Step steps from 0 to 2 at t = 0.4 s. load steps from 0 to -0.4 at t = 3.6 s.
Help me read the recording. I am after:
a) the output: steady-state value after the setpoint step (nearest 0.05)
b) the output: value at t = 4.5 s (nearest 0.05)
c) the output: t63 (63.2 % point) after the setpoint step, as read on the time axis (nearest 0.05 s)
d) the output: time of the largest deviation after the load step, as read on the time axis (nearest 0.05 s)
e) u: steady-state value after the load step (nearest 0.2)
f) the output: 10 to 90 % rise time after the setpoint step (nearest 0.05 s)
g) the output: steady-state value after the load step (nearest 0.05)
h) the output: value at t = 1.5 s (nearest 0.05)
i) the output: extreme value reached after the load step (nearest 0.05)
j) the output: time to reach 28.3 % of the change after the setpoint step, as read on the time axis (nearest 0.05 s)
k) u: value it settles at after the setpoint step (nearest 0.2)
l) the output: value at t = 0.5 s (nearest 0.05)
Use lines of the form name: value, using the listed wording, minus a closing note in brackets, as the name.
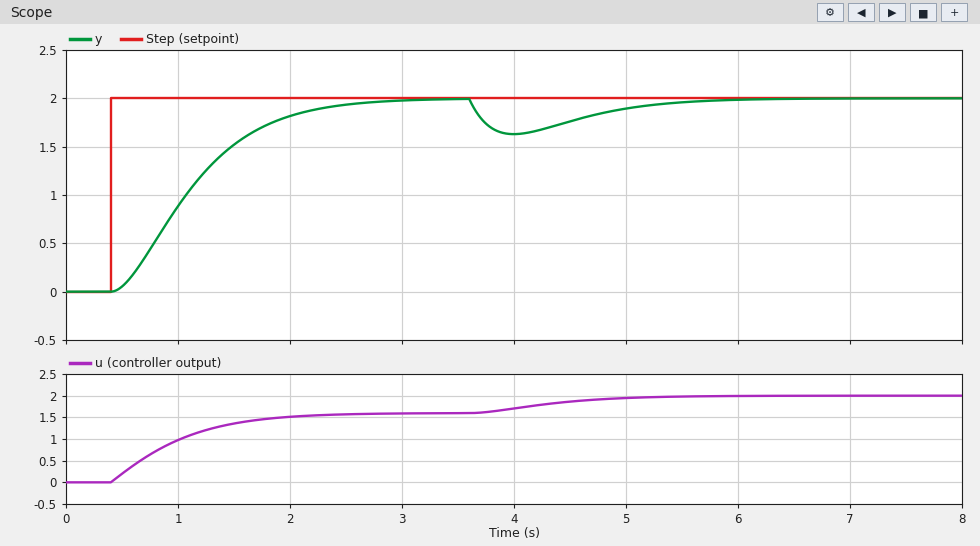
the output: steady-state value after the setpoint step: 2.00
the output: value at t = 4.5 s: 1.75
the output: t63 (63.2 % point) after the setpoint step, as read on the time axis: 1.25 s
the output: time of the largest deviation after the load step, as read on the time axis: 4.00 s
u: steady-state value after the load step: 2.0
the output: 10 to 90 % rise time after the setpoint step: 1.35 s
the output: steady-state value after the load step: 2.00
the output: value at t = 1.5 s: 1.50
the output: extreme value reached after the load step: 1.65
the output: time to reach 28.3 % of the change after the setpoint step, as read on the time axis: 0.80 s
u: value it settles at after the setpoint step: 1.6
the output: value at t = 0.5 s: 0.05
